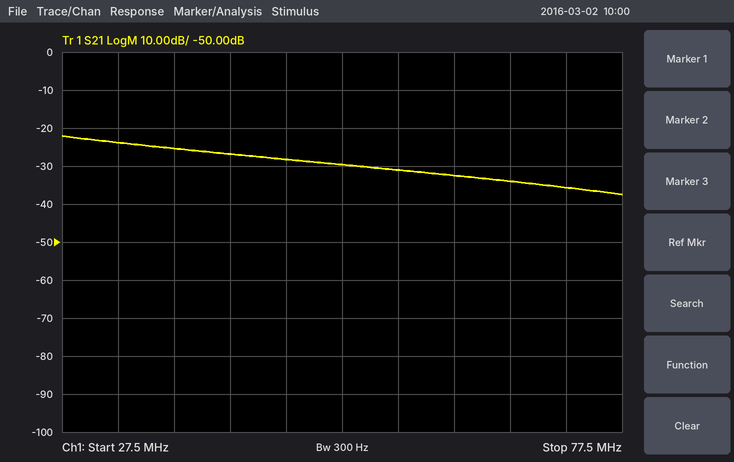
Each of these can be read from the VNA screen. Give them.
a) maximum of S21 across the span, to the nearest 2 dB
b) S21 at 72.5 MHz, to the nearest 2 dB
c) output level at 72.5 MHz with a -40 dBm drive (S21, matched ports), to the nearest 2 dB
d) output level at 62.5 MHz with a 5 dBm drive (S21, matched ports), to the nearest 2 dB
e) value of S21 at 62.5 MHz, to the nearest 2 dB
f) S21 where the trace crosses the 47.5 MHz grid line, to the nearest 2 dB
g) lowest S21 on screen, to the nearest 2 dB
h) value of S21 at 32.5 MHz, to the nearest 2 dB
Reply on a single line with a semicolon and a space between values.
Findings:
-22 dB; -36 dB; -76 dBm; -28 dBm; -32 dB; -28 dB; -38 dB; -24 dB
